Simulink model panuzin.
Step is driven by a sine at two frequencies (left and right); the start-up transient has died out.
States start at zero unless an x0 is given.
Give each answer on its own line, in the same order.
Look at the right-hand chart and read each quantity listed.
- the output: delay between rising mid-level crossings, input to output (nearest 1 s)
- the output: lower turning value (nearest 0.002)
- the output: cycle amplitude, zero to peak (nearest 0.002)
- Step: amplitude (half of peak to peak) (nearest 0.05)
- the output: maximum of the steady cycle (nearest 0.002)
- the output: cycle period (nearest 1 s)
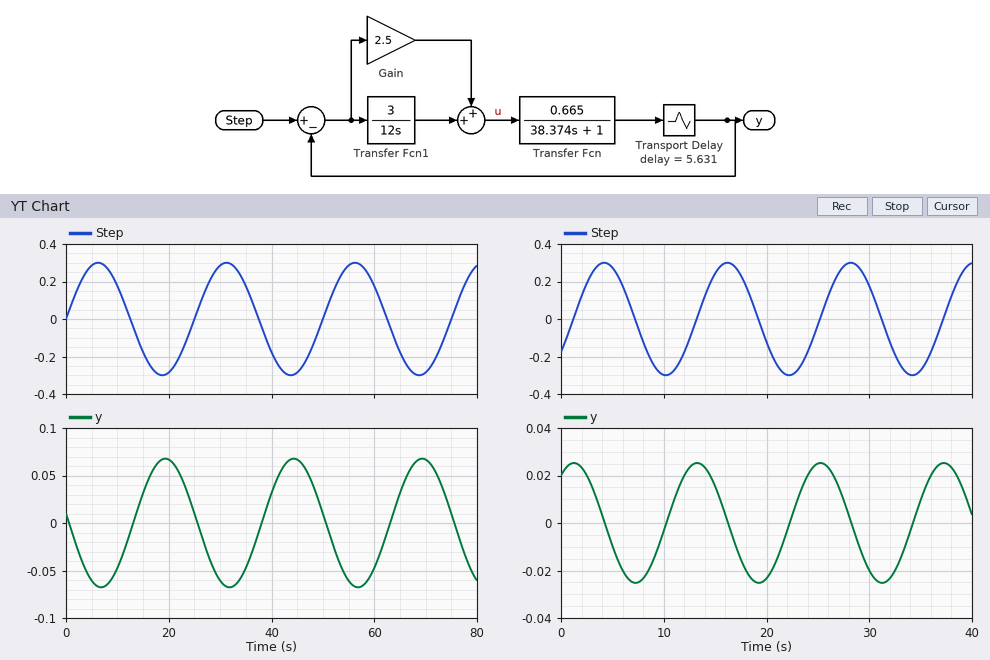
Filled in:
9 s
-0.026
0.026
0.30
0.026
12 s
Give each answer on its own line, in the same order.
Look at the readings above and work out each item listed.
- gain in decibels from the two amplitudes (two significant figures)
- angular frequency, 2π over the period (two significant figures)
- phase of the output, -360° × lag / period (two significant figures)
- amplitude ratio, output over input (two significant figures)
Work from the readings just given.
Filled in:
-21 dB
0.52 rad/s
-270°
0.087
